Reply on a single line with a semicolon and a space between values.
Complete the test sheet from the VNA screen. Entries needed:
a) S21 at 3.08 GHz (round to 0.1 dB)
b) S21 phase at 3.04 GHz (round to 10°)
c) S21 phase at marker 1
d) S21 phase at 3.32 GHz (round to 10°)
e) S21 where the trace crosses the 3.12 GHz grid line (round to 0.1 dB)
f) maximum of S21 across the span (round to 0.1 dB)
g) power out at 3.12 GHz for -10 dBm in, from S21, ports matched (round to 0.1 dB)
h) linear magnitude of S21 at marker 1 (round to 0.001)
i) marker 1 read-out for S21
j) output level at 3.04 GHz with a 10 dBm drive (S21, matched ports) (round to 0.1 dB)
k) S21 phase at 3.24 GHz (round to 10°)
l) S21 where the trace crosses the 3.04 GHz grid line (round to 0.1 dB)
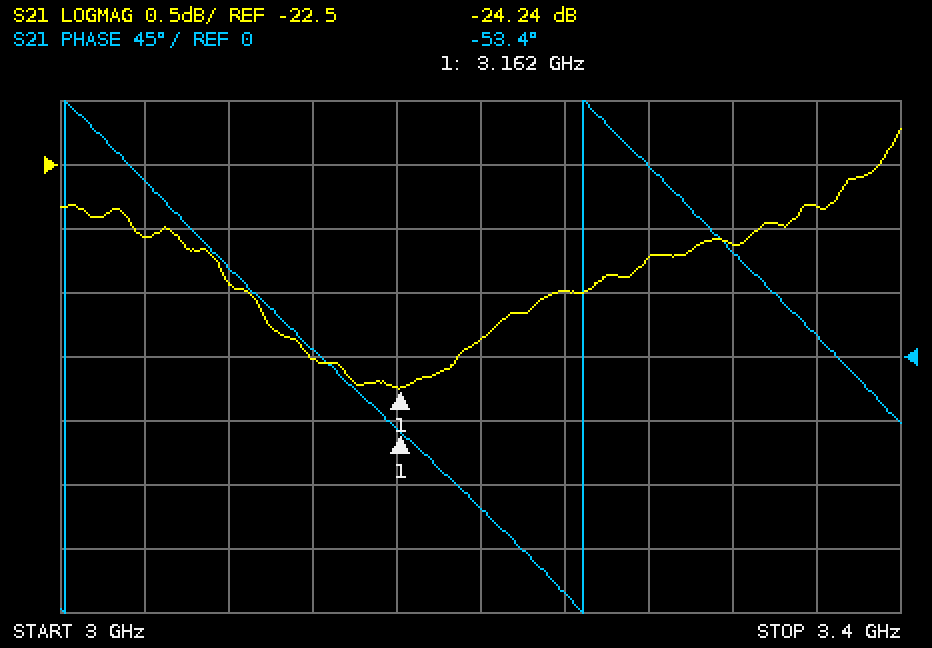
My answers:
-23.4 dB; 120°; -53.4°; 70°; -24.0 dB; -22.2 dB; -34.0 dBm; 0.061; -24.24 dB; -13.1 dBm; -170°; -23.1 dB
